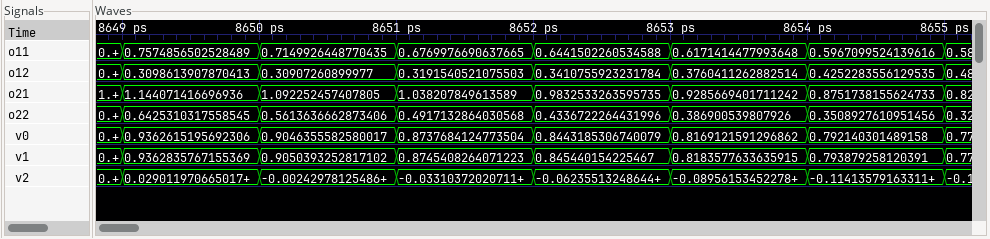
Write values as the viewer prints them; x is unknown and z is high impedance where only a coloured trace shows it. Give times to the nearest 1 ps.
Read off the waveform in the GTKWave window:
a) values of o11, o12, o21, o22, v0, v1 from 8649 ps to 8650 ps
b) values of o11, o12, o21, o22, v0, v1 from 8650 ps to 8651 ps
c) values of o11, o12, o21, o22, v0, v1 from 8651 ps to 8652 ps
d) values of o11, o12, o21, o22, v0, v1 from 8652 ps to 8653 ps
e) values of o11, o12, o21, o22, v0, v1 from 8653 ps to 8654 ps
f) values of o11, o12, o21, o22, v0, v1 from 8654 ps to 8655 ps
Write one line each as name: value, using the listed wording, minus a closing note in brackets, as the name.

values of o11, o12, o21, o22, v0, v1 from 8649 ps to 8650 ps: o11=0.7574856502528489, o12=0.3098613907870413, o21=1.144071416696936, o22=0.6425310317558545, v0=0.9362615195692306, v1=0.9362835767155369
values of o11, o12, o21, o22, v0, v1 from 8650 ps to 8651 ps: o11=0.7149926448770435, o12=0.30907260899977, o21=1.092252457407805, o22=0.5613636662873406, v0=0.9046355582580017, v1=0.9050393252817102
values of o11, o12, o21, o22, v0, v1 from 8651 ps to 8652 ps: o11=0.6769976690637665, o12=0.3191540521075503, o21=1.038207849613589, o22=0.4917132864030568, v0=0.8737684124773504, v1=0.8745408264071223
values of o11, o12, o21, o22, v0, v1 from 8652 ps to 8653 ps: o11=0.6441502260534588, o12=0.3410755923231784, o21=0.9832533263595735, o22=0.4336722264431996, v0=0.8443185306740079, v1=0.845440154225467
values of o11, o12, o21, o22, v0, v1 from 8653 ps to 8654 ps: o11=0.6171414477993648, o12=0.3760411262882514, o21=0.9285669401711242, o22=0.386900539807926, v0=0.8169121591296862, v1=0.8183577633635915
values of o11, o12, o21, o22, v0, v1 from 8654 ps to 8655 ps: o11=0.5967099524139616, o12=0.4252283556129535, o21=0.8751738155624733, o22=0.3508927610951456, v0=0.792140301489158, v1=0.793879258120391
